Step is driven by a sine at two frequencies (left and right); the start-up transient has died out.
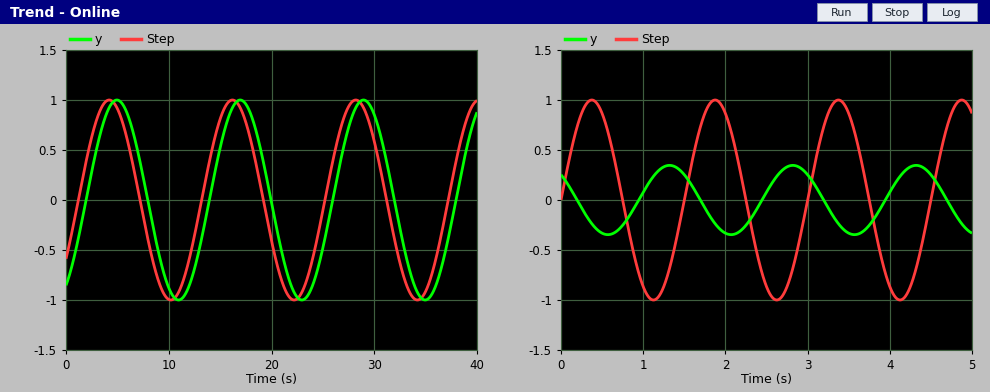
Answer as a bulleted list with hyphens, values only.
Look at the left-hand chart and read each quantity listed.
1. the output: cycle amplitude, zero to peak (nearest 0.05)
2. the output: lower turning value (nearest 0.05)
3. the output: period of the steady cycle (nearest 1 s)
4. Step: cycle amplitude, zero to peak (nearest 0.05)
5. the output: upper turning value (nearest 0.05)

- 1.00
- -1.00
- 12 s
- 1.00
- 1.00
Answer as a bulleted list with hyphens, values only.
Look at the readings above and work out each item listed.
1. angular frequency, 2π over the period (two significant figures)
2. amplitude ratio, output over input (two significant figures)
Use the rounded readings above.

- 0.52 rad/s
- 1.0
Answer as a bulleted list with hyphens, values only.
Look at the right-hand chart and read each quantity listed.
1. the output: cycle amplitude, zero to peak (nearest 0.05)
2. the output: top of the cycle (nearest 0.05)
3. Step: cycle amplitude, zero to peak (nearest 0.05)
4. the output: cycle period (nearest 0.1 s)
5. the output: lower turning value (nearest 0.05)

- 0.35
- 0.35
- 1.00
- 1.5 s
- -0.35
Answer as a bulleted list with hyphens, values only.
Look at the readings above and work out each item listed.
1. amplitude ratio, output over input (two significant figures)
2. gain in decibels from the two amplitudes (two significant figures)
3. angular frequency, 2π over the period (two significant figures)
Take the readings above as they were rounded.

- 0.35
- -9.1 dB
- 4.2 rad/s
